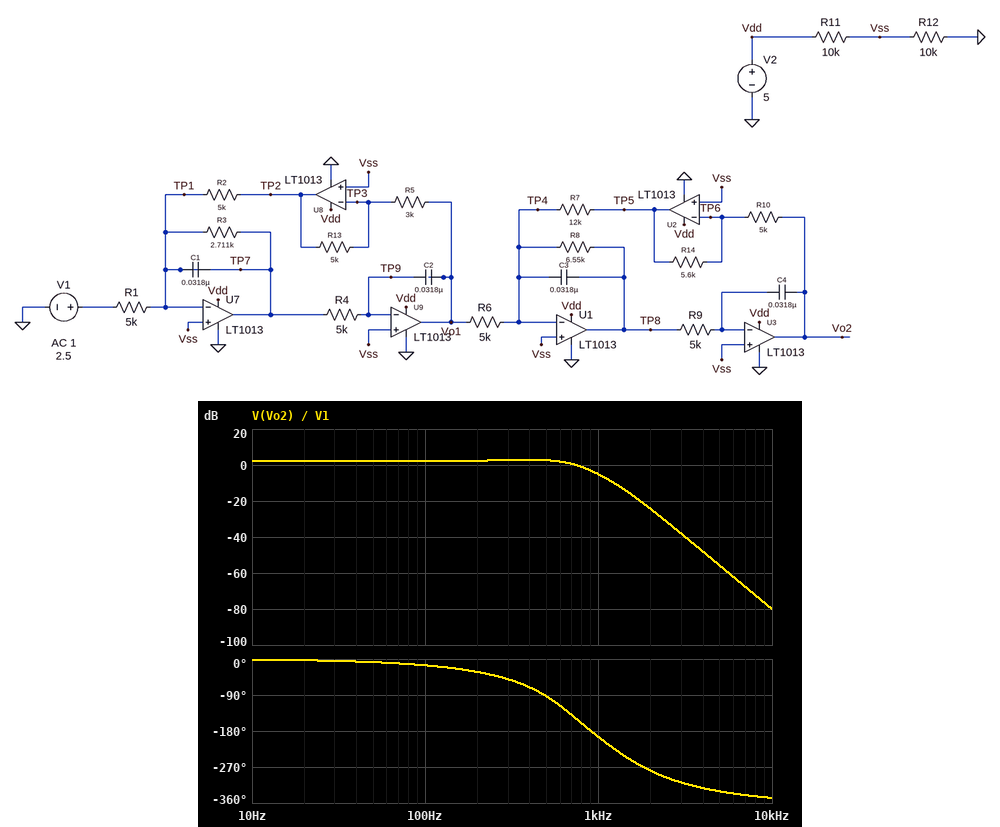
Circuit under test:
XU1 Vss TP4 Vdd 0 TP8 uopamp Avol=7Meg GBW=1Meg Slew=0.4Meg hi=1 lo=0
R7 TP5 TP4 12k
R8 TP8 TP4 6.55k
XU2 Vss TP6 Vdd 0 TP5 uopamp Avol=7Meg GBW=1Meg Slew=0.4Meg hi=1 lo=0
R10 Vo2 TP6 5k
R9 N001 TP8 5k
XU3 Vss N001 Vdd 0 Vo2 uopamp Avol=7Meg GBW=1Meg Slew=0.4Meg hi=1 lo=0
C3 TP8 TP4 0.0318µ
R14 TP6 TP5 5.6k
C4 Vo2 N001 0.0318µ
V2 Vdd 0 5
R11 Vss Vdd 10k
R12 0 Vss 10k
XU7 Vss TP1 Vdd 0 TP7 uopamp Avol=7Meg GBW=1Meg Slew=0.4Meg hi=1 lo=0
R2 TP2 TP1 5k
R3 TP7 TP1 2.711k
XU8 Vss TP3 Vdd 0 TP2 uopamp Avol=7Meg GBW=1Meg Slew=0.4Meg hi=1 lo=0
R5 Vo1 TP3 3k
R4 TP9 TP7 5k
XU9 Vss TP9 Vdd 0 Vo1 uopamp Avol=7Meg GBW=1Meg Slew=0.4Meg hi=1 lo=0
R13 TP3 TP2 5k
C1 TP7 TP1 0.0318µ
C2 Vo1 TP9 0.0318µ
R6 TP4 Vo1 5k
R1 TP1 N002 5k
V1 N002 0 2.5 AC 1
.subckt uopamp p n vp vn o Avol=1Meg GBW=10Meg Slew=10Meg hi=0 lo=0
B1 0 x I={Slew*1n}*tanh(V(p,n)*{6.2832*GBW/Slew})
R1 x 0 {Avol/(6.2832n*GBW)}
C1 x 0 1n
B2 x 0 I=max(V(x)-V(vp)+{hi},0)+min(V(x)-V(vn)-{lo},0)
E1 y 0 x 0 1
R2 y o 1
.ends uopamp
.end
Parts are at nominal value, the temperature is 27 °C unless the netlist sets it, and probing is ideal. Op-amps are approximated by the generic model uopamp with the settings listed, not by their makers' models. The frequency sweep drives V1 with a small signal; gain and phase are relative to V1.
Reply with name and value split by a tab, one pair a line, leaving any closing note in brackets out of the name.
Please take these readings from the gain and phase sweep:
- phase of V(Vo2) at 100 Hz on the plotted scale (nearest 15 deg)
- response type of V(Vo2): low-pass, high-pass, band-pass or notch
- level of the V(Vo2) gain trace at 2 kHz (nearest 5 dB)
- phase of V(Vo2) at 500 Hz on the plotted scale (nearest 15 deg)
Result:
phase of V(Vo2) at 100 Hz on the plotted scale	-15 deg
response type of V(Vo2): low-pass, high-pass, band-pass or notch	low-pass
level of the V(Vo2) gain trace at 2 kHz	-25 dB
phase of V(Vo2) at 500 Hz on the plotted scale	-90 deg
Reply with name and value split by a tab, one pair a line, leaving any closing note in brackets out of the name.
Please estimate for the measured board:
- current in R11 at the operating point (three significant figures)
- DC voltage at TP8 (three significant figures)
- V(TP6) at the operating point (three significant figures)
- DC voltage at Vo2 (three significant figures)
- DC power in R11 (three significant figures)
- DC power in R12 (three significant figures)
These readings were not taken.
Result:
current in R11 at the operating point	250 µA
DC voltage at TP8	2.50 V
V(TP6) at the operating point	2.50 V
DC voltage at Vo2	2.50 V
DC power in R11	625 µW
DC power in R12	625 µW
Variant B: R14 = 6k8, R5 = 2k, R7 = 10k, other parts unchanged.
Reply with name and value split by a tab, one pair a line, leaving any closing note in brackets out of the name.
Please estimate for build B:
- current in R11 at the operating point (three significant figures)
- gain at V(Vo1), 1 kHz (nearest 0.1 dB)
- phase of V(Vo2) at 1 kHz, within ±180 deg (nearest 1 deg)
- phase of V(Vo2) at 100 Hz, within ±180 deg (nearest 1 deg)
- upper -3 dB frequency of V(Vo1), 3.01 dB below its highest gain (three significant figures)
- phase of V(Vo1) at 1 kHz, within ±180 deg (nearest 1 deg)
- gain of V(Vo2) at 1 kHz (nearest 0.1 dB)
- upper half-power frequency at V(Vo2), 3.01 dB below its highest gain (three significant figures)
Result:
current in R11 at the operating point	250 µA
gain at V(Vo1), 1 kHz	-7.5 dB
phase of V(Vo2) at 1 kHz, within ±180 deg	-164 deg
phase of V(Vo2) at 100 Hz, within ±180 deg	-11 deg
upper -3 dB frequency of V(Vo1), 3.01 dB below its highest gain	1.78 kHz
phase of V(Vo1) at 1 kHz, within ±180 deg	-51 deg
gain of V(Vo2) at 1 kHz	-5.8 dB
upper half-power frequency at V(Vo2), 3.01 dB below its highest gain	981 Hz
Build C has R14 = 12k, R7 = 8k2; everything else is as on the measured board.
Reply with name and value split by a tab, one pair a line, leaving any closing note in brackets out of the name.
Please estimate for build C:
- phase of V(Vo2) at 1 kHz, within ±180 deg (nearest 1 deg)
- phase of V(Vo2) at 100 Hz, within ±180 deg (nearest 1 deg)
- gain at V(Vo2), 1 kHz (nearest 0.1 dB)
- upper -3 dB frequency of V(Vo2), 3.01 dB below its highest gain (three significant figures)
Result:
phase of V(Vo2) at 1 kHz, within ±180 deg	-129 deg
phase of V(Vo2) at 100 Hz, within ±180 deg	-9 deg
gain at V(Vo2), 1 kHz	-4.8 dB
upper -3 dB frequency of V(Vo2), 3.01 dB below its highest gain	1.31 kHz
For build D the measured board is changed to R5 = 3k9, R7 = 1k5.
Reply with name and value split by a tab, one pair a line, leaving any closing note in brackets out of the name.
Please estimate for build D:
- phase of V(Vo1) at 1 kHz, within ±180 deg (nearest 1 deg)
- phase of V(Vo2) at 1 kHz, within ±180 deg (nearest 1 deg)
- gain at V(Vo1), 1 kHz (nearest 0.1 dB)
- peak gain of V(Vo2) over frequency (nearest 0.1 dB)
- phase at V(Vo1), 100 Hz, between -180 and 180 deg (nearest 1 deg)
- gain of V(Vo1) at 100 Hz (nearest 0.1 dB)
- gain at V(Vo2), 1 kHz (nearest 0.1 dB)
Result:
phase of V(Vo1) at 1 kHz, within ±180 deg	-81 deg
phase of V(Vo2) at 1 kHz, within ±180 deg	-97 deg
gain at V(Vo1), 1 kHz	-5.4 dB
peak gain of V(Vo2) over frequency	-13.6 dB
phase at V(Vo1), 100 Hz, between -180 and 180 deg	-8 deg
gain of V(Vo1) at 100 Hz	-2.2 dB
gain at V(Vo2), 1 kHz	-14.4 dB
